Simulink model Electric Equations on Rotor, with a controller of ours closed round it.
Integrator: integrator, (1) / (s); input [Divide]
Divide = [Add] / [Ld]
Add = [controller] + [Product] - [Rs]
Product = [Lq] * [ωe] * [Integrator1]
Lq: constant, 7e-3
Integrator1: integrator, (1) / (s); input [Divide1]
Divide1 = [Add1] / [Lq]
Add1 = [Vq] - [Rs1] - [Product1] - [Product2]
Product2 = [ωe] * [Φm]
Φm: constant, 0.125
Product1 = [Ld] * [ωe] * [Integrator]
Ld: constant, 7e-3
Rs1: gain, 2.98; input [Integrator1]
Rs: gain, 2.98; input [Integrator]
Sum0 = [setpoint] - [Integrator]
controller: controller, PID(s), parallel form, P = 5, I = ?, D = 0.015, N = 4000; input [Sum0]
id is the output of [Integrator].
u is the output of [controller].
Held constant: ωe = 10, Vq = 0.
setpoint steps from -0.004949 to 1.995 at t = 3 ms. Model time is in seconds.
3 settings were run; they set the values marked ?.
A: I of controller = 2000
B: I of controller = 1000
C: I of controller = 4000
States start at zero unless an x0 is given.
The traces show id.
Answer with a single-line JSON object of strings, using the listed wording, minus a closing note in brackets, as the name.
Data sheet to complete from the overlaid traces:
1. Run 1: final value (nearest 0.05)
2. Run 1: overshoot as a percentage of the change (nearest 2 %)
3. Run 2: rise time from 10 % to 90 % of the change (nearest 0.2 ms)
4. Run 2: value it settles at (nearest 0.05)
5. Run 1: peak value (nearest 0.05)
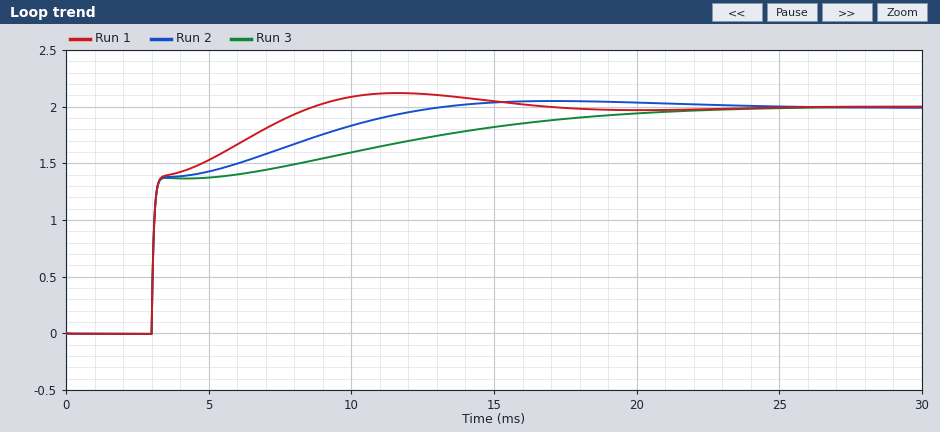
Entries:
{"Run 1: final value": "2.00", "Run 1: overshoot as a percentage of the change": "6 %", "Run 2: rise time from 10 % to 90 % of the change": "6.4 ms", "Run 2: value it settles at": "2.00", "Run 1: peak value": "2.10"}
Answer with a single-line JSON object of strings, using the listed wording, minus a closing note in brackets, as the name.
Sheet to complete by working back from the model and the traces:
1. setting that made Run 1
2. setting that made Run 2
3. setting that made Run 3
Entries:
{"setting that made Run 1": "C", "setting that made Run 2": "A", "setting that made Run 3": "B"}
